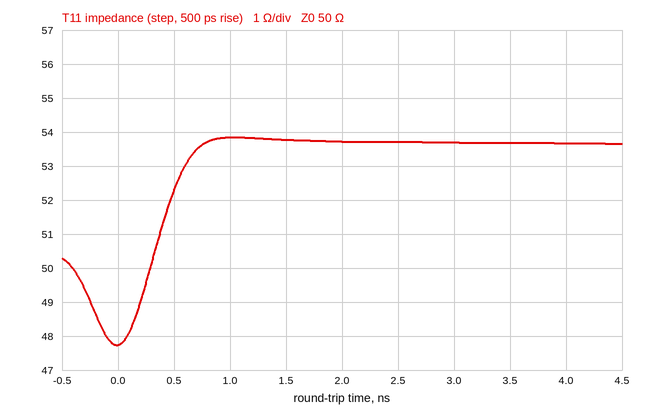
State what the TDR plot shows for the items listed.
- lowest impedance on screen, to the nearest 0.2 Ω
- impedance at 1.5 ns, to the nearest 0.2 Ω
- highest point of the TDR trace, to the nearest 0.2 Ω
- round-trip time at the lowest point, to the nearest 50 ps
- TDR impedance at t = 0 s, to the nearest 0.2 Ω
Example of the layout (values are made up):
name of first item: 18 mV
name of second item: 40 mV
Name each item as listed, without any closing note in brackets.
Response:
lowest impedance on screen, to the nearest 0.2 Ω: 47.8 Ω
impedance at 1.5 ns, to the nearest 0.2 Ω: 53.8 Ω
highest point of the TDR trace, to the nearest 0.2 Ω: 53.8 Ω
round-trip time at the lowest point, to the nearest 50 ps: 0 ps
TDR impedance at t = 0 s, to the nearest 0.2 Ω: 47.8 Ω
